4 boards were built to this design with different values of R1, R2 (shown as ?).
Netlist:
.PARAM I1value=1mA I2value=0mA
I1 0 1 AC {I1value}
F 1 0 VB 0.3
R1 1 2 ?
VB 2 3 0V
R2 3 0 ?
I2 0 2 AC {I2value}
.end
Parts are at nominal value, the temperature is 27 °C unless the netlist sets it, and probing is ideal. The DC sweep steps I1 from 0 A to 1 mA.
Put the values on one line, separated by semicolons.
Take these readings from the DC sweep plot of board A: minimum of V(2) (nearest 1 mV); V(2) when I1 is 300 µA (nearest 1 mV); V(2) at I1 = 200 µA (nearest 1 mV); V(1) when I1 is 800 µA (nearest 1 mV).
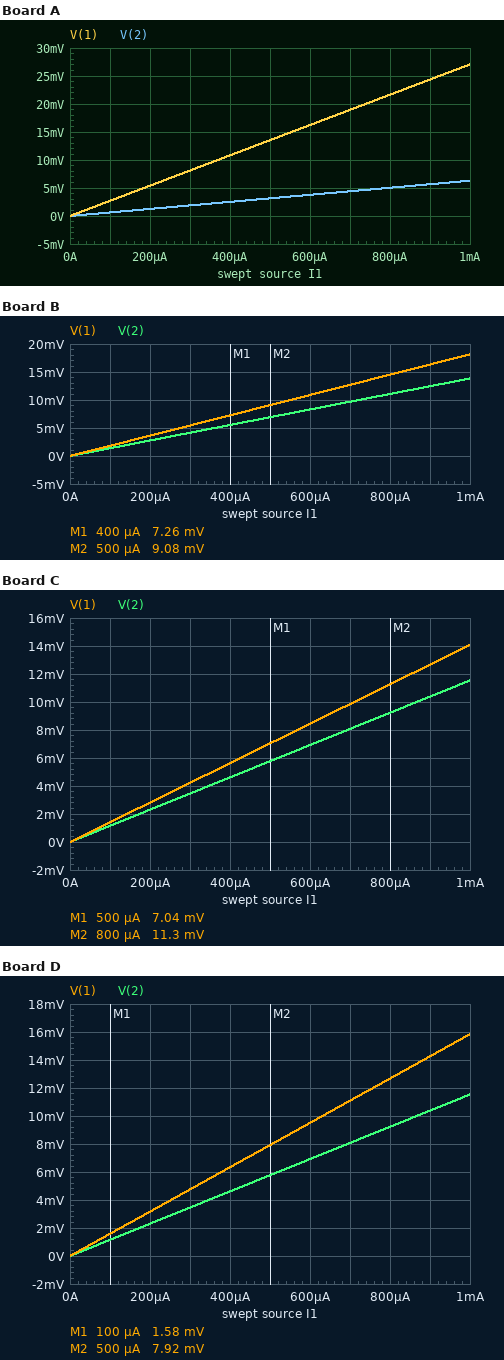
0 V; 2 mV; 1 mV; 22 mV
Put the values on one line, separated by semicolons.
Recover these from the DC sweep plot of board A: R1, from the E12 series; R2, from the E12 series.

27 Ω; 8.2 Ω
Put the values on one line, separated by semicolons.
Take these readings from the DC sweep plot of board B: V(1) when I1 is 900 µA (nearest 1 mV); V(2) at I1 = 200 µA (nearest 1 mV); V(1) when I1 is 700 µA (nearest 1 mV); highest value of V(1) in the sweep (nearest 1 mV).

16 mV; 3 mV; 13 mV; 18 mV
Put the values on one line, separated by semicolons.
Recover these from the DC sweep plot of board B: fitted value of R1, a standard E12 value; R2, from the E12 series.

5.6 Ω; 18 Ω
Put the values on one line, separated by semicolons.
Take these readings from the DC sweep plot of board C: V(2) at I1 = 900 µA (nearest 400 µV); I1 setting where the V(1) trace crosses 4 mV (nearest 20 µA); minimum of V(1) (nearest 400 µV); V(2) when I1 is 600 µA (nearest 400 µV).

10.4 mV; 280 µA; 0 V; 6.8 mV
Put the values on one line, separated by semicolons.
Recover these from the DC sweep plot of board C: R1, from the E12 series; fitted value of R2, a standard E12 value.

3.3 Ω; 15 Ω
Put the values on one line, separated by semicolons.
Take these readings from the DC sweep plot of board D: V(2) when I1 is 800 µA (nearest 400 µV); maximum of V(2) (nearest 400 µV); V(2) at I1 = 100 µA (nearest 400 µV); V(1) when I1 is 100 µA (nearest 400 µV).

9.2 mV; 11.6 mV; 1.2 mV; 1.6 mV
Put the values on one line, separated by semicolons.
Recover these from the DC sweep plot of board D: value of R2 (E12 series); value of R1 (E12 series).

15 Ω; 5.6 Ω
